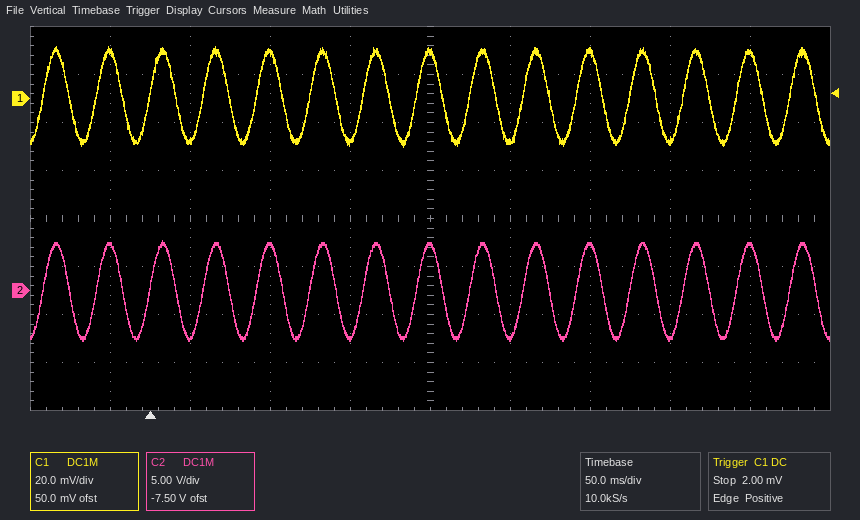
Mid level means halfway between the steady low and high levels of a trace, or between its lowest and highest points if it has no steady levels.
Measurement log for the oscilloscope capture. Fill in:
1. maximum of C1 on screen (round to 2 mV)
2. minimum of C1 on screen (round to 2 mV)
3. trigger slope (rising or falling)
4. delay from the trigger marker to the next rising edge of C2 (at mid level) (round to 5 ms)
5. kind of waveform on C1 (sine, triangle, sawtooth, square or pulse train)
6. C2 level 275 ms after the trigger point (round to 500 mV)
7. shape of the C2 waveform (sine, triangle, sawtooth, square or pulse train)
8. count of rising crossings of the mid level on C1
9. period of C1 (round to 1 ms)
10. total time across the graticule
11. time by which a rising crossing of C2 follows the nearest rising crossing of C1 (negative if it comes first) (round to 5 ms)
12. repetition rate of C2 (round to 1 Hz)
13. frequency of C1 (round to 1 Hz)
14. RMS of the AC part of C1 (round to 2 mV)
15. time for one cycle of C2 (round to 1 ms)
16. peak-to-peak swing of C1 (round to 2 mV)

22 mV
-20 mV
rising
35 ms
sine
4.5 V
sine
15
33 ms
500 ms
0 ms
30 Hz
30 Hz
14 mV
33 ms
42 mV
